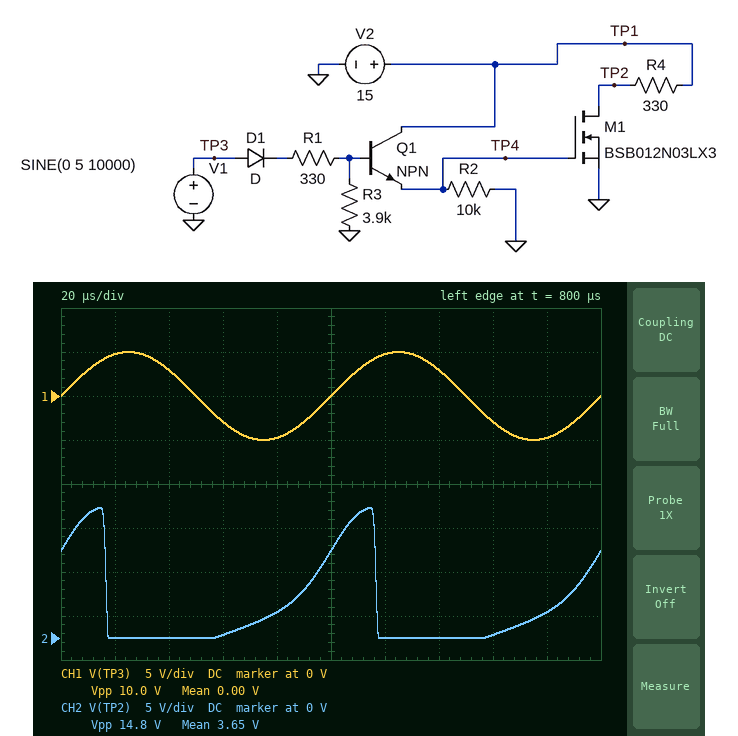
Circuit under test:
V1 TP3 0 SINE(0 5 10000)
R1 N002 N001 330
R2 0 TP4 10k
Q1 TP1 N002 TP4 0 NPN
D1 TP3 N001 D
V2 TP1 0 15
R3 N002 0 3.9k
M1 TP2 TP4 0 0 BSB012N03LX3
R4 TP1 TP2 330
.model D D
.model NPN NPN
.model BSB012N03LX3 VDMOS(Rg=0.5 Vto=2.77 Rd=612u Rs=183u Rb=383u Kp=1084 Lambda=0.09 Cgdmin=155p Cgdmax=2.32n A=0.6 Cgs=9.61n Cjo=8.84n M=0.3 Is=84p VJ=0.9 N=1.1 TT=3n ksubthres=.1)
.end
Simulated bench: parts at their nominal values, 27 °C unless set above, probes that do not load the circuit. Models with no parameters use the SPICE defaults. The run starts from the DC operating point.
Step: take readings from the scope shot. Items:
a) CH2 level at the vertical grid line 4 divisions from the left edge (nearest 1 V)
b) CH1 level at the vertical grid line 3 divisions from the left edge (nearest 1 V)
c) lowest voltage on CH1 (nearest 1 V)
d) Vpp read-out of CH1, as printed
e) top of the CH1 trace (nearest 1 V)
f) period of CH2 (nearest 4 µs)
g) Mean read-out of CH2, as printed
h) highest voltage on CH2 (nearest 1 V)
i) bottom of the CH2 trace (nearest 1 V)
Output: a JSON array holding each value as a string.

["3 V", "-3 V", "-5 V", "10.0 V", "5 V", "100 µs", "3.65 V", "15 V", "0 V"]
